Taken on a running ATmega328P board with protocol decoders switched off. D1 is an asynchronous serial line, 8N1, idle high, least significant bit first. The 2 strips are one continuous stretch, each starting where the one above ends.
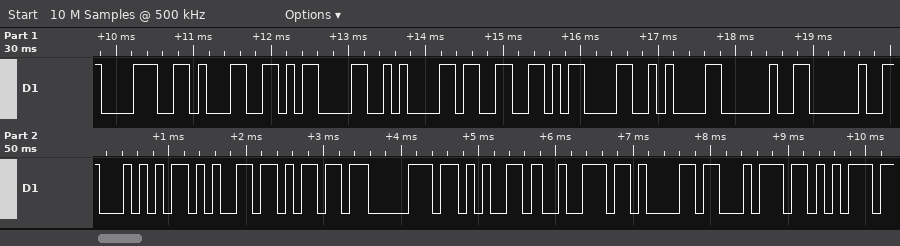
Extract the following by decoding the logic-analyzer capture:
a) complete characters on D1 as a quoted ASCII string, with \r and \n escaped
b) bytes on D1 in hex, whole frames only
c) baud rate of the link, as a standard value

"81\r\n3\r\n  Temperatu"
0x38 0x31 0x0D 0x0A 0x33 0x0D 0x0A 0x20 0x20 0x54 0x65 0x6D 0x70 0x65 0x72 0x61 0x74 0x75
9600 baud
